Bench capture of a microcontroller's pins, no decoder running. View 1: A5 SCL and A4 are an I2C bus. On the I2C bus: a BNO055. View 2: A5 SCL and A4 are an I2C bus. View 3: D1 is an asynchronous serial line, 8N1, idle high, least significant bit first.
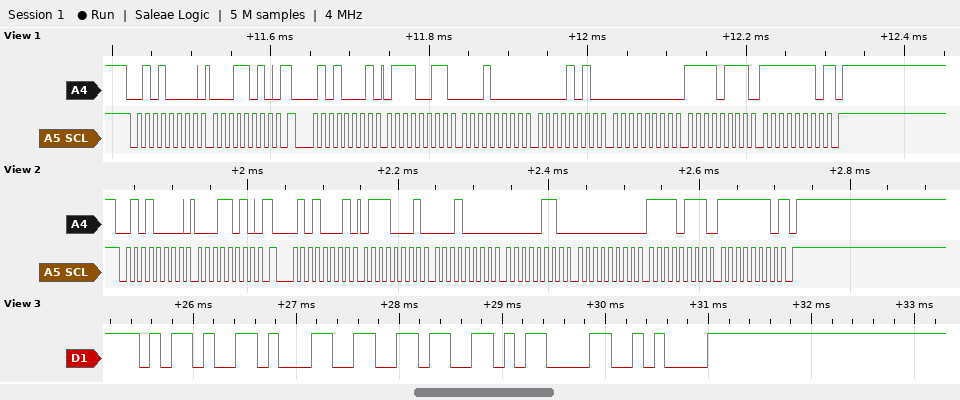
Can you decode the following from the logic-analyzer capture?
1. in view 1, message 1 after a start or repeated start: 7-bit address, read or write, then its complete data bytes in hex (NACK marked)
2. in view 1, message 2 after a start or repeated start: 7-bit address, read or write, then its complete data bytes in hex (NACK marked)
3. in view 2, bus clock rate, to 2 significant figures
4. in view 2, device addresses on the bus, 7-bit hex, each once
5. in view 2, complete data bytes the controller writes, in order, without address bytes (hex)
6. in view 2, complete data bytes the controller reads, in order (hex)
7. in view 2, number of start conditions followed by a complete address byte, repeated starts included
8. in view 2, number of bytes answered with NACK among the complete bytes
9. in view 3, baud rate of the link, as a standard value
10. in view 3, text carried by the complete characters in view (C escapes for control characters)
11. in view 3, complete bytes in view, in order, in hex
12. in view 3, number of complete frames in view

0x28 write: 1A
0x28 read: 73 10 0A 00 F7 FE NACK
100 kHz
0x28
1A
71 10 06 00 F7 FE
2
1
9600 baud
"-16\r\n"
0x2D 0x31 0x36 0x0D 0x0A
5
